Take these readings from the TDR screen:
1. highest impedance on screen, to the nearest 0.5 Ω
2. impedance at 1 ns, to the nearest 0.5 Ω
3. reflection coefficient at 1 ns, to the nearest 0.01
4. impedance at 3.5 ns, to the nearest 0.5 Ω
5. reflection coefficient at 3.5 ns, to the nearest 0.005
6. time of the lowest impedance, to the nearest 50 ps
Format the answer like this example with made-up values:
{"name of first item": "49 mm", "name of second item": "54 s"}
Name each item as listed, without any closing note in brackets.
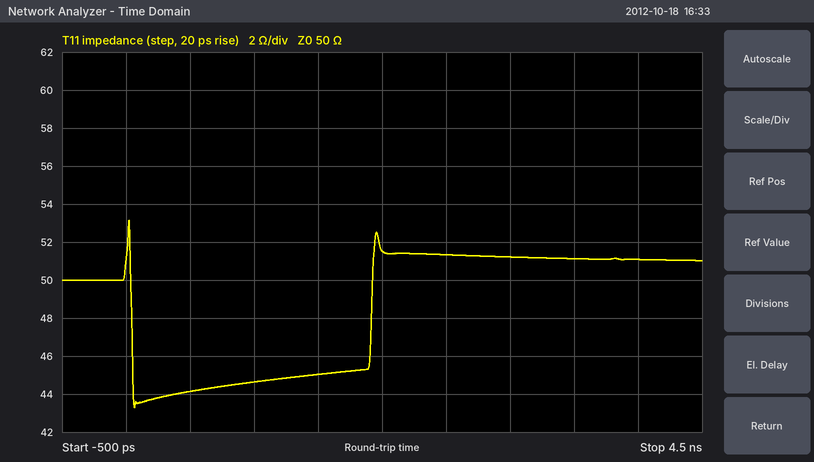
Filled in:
{"highest impedance on screen, to the nearest 0.5 Ω": "53.0 Ω", "impedance at 1 ns, to the nearest 0.5 Ω": "44.5 Ω", "reflection coefficient at 1 ns, to the nearest 0.01": "-0.06", "impedance at 3.5 ns, to the nearest 0.5 Ω": "51.0 Ω", "reflection coefficient at 3.5 ns, to the nearest 0.005": "+0.010", "time of the lowest impedance, to the nearest 50 ps": "50 ps"}
